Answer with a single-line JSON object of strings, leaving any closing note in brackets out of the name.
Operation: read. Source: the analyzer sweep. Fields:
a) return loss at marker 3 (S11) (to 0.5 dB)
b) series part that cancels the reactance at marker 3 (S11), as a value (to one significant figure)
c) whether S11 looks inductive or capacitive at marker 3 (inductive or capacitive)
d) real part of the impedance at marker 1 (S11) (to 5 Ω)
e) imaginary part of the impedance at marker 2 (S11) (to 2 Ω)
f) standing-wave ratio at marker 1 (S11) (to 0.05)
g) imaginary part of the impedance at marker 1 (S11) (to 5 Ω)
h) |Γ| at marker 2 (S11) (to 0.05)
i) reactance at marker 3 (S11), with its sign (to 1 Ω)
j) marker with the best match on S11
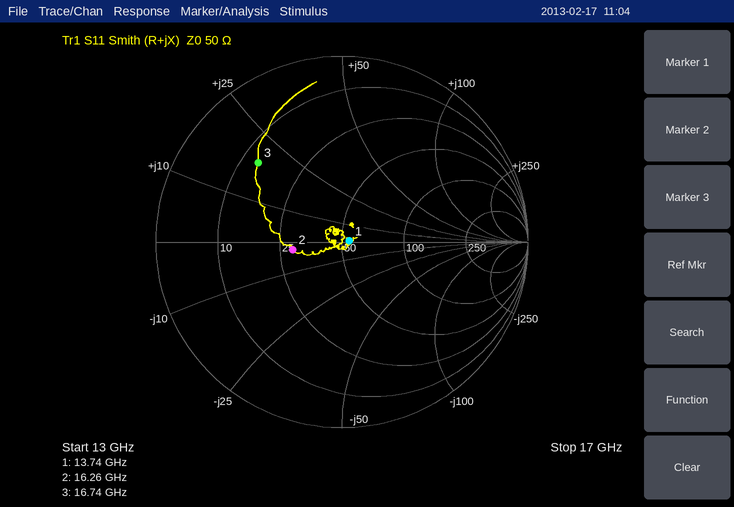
{"return loss at marker 3 (S11)": "4.0 dB", "series part that cancels the reactance at marker 3 (S11), as a value": "500 fF", "whether S11 looks inductive or capacitive at marker 3": "inductive", "real part of the impedance at marker 1 (S11)": "55 Ω", "imaginary part of the impedance at marker 2 (S11)": "-2 Ω", "standing-wave ratio at marker 1 (S11)": "1.10", "imaginary part of the impedance at marker 1 (S11)": "0 Ω", "|Γ| at marker 2 (S11)": "0.25", "reactance at marker 3 (S11), with its sign": "+19 Ω", "marker with the best match on S11": "marker 1"}
